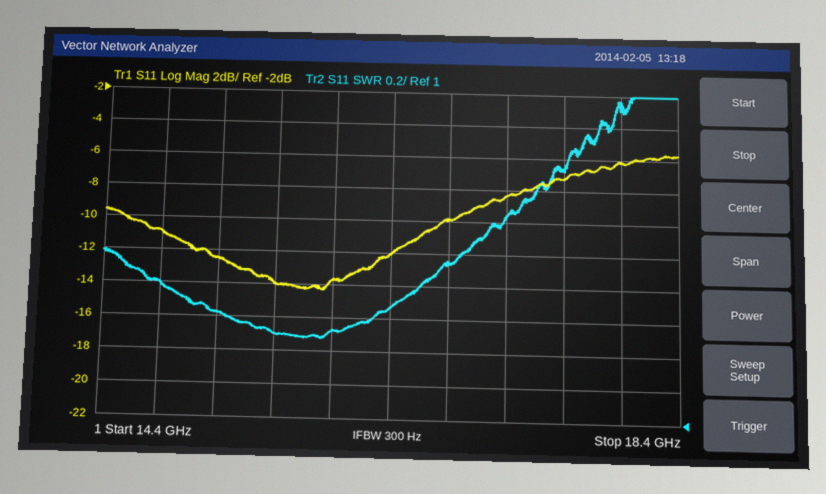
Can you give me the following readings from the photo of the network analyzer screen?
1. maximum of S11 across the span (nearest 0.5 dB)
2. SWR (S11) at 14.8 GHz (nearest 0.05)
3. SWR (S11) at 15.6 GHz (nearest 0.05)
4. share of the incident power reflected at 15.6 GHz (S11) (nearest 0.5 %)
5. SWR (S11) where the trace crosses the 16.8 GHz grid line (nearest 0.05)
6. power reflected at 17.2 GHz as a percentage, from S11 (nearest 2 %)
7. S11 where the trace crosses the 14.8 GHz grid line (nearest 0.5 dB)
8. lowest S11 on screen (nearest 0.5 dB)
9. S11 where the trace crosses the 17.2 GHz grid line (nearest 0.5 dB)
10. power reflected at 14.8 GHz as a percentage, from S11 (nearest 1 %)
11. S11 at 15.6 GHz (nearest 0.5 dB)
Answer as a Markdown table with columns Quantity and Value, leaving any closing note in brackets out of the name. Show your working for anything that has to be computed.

| Quantity | Value |
|---|---|
| maximum of S11 across the span | -5.5 dB |
| SWR (S11) at 14.8 GHz | 1.80 |
| SWR (S11) at 15.6 GHz | 1.50 |
| share of the incident power reflected at 15.6 GHz (S11) | 10^(-14/10) ≈ 4.0 % |
| SWR (S11) where the trace crosses the 16.8 GHz grid line | 1.95 |
| power reflected at 17.2 GHz as a percentage, from S11 | 10^(-8.5/10) ≈ 14 % |
| S11 where the trace crosses the 14.8 GHz grid line | -11.0 dB |
| lowest S11 on screen | -14.5 dB |
| S11 where the trace crosses the 17.2 GHz grid line | -8.5 dB |
| power reflected at 14.8 GHz as a percentage, from S11 | 10^(-11/10) ≈ 8 % |
| S11 at 15.6 GHz | -14.0 dB |
